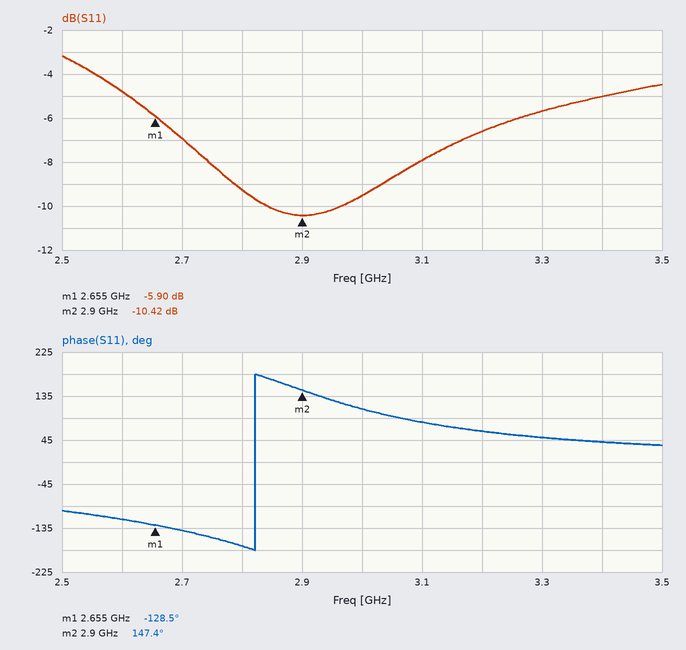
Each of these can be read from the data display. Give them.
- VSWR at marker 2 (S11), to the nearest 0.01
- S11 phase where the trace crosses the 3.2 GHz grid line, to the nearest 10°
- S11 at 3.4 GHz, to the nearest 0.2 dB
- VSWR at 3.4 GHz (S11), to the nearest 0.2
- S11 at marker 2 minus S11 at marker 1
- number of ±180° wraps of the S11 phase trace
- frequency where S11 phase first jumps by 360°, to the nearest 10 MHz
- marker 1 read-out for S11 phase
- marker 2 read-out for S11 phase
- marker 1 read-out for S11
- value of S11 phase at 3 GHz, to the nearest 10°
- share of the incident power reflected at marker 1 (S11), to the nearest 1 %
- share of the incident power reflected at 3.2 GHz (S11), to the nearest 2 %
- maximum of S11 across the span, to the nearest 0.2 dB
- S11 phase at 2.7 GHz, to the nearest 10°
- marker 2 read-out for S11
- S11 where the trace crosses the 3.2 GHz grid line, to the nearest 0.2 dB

1.86
60°
-5.0 dB
3.6
-4.52 dB
1
2.82 GHz
-128.5°
147.4°
-5.90 dB
110°
26 %
22 %
-3.2 dB
-140°
-10.42 dB
-6.6 dB
